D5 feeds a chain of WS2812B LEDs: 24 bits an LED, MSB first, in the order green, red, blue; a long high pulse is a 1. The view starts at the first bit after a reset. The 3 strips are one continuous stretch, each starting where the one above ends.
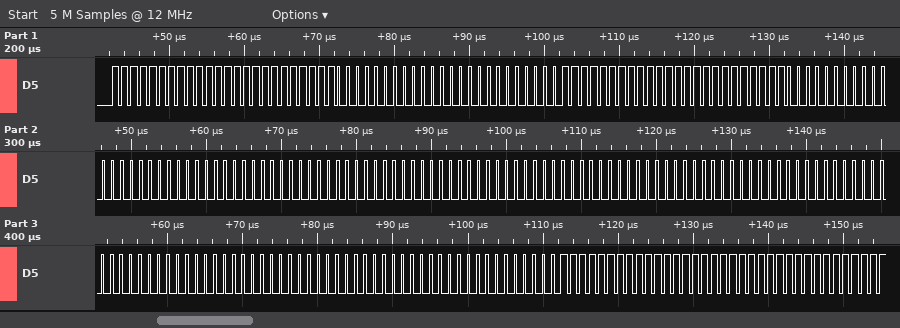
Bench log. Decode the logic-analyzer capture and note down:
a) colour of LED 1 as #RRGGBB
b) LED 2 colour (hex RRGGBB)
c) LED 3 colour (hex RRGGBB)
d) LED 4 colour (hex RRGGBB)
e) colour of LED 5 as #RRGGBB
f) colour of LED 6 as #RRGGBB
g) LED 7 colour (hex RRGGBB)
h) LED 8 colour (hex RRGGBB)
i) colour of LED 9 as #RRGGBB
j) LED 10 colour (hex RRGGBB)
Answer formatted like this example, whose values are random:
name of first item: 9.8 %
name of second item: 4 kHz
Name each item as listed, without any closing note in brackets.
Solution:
colour of LED 1 as #RRGGBB: #FFFFFF
LED 2 colour: #000000
LED 3 colour: #FFFFFF
LED 4 colour: #000000
colour of LED 5 as #RRGGBB: #000000
colour of LED 6 as #RRGGBB: #000000
LED 7 colour: #000000
LED 8 colour: #000000
colour of LED 9 as #RRGGBB: #000000
LED 10 colour: #FFFFFF
